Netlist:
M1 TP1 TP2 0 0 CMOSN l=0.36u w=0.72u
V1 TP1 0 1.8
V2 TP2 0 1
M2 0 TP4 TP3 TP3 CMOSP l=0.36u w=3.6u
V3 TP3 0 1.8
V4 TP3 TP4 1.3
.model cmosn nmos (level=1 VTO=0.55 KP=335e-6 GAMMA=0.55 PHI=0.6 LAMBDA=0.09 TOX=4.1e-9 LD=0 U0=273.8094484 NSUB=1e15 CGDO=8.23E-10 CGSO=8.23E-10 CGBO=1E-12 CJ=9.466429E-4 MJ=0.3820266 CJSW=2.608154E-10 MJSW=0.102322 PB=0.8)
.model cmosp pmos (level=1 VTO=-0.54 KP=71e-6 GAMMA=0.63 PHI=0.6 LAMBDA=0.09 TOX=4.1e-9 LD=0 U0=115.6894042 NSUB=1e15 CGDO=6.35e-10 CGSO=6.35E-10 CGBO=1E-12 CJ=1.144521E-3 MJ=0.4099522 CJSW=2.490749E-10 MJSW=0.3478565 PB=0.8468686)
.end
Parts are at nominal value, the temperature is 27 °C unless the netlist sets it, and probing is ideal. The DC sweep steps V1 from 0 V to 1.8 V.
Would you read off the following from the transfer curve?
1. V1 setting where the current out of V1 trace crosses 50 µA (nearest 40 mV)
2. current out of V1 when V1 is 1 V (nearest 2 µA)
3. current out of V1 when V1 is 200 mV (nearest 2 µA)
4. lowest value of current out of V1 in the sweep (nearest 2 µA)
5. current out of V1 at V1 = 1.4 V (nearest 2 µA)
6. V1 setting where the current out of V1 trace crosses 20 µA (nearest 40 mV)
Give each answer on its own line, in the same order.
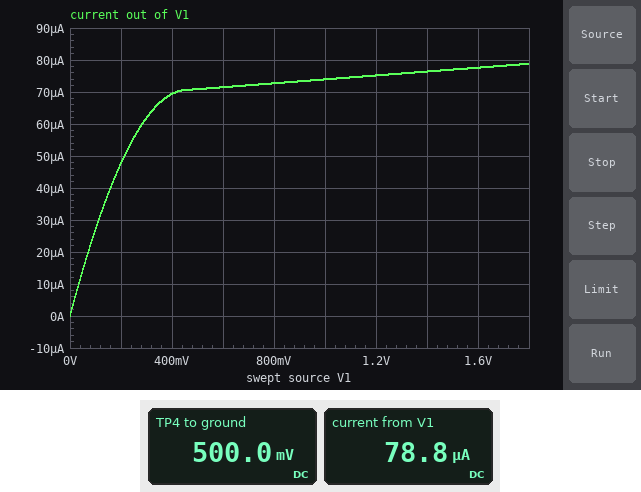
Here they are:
200 mV
74 µA
48 µA
0 A
76 µA
80 mV
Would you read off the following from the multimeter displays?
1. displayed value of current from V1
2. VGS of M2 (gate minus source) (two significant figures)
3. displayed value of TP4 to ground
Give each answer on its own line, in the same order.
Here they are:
78.8 µA
-1.3 V
500.0 mV
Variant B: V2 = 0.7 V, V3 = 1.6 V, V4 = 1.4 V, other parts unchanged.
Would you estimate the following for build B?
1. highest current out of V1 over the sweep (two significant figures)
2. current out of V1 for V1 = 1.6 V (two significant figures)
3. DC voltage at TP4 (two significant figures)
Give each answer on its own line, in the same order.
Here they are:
8.8 µA
8.6 µA
200 mV
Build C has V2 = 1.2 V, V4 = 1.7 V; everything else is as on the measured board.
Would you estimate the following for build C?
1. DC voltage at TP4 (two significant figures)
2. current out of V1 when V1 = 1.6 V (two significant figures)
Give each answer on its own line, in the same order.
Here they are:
100 mV
160 µA
